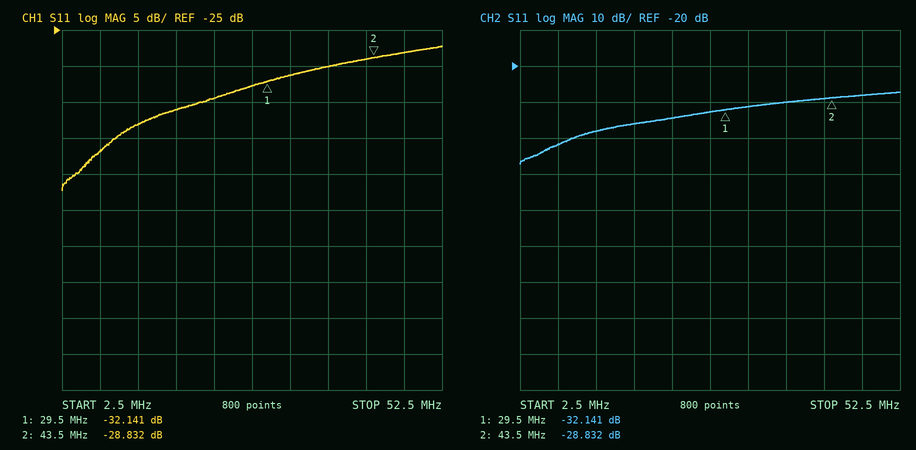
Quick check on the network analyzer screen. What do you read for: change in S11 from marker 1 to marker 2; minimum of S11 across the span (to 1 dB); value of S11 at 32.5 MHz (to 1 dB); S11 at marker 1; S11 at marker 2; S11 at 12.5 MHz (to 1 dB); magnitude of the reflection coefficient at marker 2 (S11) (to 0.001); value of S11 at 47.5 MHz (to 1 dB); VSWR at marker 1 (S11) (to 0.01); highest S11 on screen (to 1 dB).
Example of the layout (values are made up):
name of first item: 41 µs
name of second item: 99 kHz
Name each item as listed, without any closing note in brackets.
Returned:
change in S11 from marker 1 to marker 2: 3.309 dB
minimum of S11 across the span: -47 dB
value of S11 at 32.5 MHz: -31 dB
S11 at marker 1: -32.141 dB
S11 at marker 2: -28.832 dB
S11 at 12.5 MHz: -38 dB
magnitude of the reflection coefficient at marker 2 (S11): 0.036
value of S11 at 47.5 MHz: -28 dB
VSWR at marker 1 (S11): 1.05
highest S11 on screen: -27 dB
